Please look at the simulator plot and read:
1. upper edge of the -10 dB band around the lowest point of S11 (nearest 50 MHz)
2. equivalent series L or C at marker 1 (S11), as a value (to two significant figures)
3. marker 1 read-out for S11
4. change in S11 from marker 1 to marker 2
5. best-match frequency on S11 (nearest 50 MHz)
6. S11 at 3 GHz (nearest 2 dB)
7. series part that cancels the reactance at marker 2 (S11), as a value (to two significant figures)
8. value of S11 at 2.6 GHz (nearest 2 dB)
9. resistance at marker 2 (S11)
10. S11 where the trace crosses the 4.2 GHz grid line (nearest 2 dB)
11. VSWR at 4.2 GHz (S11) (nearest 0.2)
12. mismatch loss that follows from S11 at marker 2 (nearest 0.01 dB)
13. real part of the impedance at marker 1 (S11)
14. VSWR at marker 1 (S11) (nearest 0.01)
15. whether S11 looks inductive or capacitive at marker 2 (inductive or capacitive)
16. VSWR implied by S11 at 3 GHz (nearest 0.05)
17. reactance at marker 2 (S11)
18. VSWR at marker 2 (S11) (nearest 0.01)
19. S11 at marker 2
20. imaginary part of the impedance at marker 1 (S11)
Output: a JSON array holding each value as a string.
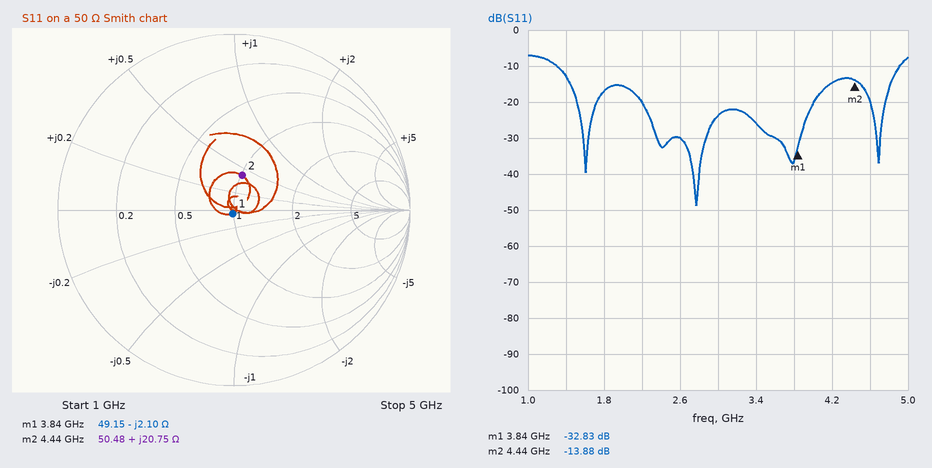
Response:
["4.90 GHz", "20 pF", "-32.83 dB", "18.95 dB", "2.75 GHz", "-24 dB", "1.7 pF", "-30 dB", "50.48 Ω", "-14 dB", "1.4", "0.18 dB", "49.15 Ω", "1.05", "inductive", "1.15", "+20.75 Ω", "1.51", "-13.88 dB", "-2.10 Ω"]
